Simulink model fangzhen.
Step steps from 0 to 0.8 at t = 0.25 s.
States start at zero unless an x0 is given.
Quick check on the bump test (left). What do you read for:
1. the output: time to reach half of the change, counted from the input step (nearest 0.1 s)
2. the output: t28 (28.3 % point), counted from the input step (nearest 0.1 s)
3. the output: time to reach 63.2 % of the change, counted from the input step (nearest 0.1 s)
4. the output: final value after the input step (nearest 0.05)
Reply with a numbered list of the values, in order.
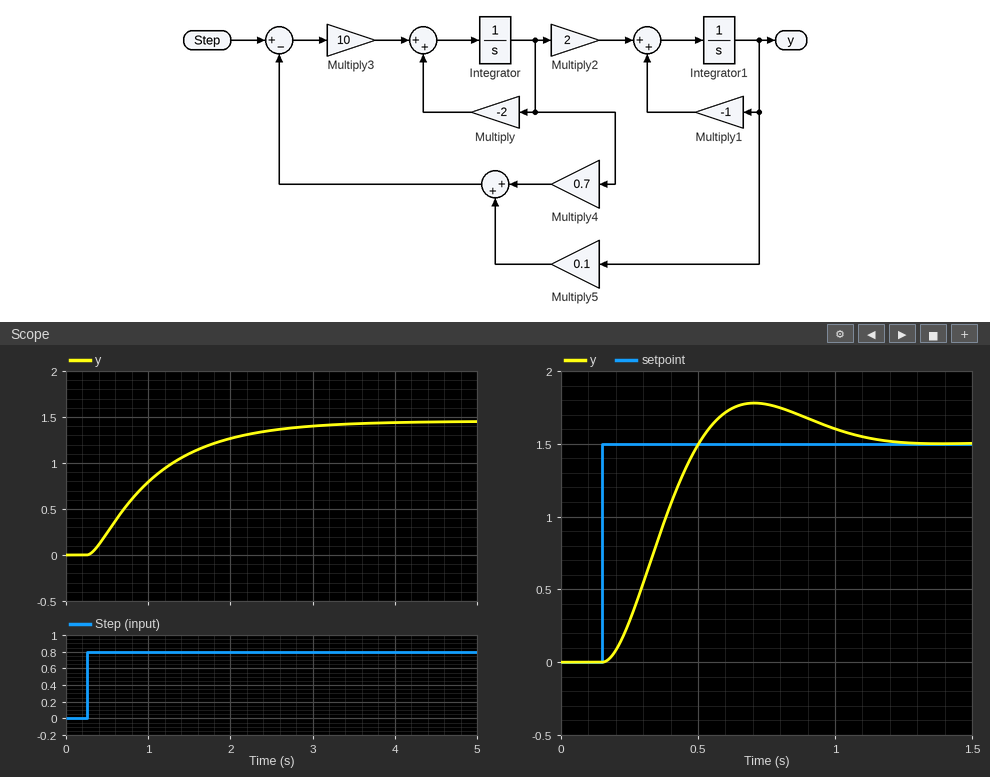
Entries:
1. 0.7 s
2. 0.4 s
3. 0.9 s
4. 1.45
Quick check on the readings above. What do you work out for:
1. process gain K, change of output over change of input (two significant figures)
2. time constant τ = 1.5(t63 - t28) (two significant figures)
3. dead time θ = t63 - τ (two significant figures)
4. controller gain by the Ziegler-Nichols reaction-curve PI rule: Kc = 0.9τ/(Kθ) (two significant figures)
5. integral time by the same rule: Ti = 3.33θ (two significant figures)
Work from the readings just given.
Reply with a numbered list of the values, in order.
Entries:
1. 1.8
2. 0.75 s
3. 0.15 s
4. 2.5
5. 0.50 s
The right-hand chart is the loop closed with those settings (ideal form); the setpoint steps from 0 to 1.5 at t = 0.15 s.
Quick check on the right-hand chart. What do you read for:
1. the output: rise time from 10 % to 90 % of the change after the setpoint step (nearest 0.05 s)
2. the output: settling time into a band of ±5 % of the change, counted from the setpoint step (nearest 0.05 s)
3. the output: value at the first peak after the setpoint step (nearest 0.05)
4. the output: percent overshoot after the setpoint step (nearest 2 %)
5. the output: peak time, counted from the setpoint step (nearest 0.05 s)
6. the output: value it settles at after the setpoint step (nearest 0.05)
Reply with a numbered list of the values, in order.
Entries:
1. 0.25 s
2. 0.90 s
3. 1.80
4. 18 %
5. 0.55 s
6. 1.50
